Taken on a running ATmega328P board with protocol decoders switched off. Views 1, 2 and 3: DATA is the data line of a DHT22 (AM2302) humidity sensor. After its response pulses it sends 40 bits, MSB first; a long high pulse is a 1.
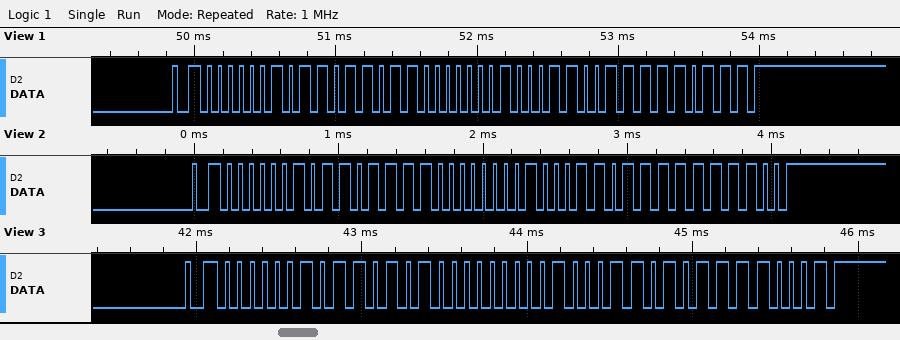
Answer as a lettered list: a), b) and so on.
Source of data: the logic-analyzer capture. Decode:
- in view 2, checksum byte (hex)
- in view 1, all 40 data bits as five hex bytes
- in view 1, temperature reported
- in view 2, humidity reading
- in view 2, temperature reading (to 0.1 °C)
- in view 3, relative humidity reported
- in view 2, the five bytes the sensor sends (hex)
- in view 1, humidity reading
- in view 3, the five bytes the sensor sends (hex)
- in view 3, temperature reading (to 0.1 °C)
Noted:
a) 0xFC
b) 02 DB 01 19 F7
c) 28.1 °C
d) 73.4 %
e) 28.3 °C
f) 72.4 %
g) 02 DE 01 1B FC
h) 73.1 %
i) 02 D4 01 1A F1
j) 28.2 °C
